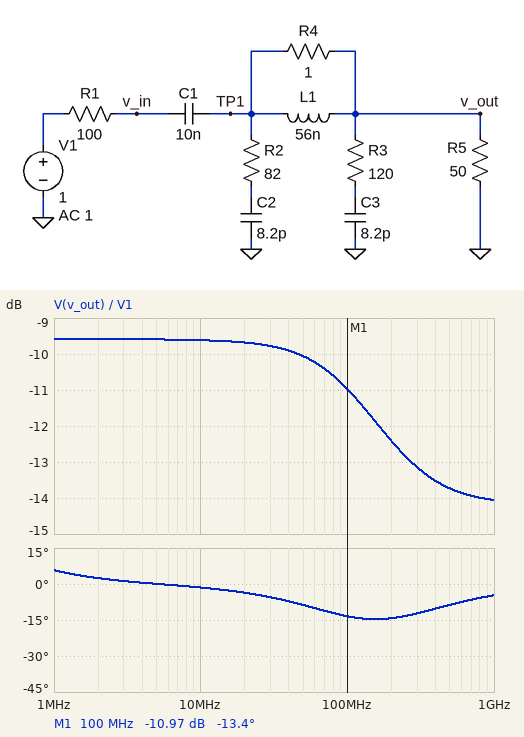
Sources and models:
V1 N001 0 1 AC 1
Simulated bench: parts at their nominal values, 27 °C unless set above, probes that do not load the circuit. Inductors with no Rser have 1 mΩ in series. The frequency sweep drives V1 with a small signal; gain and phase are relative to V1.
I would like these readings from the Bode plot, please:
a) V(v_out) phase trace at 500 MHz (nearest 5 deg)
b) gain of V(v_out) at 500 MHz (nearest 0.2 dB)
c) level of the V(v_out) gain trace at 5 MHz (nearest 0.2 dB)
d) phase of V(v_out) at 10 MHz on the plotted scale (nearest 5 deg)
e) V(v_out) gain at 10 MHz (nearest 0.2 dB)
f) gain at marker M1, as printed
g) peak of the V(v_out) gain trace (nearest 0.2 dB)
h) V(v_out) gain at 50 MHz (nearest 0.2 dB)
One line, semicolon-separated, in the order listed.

-10 deg; -13.8 dB; -9.6 dB; 0 deg; -9.6 dB; -10.97 dB; -9.6 dB; -10.0 dB
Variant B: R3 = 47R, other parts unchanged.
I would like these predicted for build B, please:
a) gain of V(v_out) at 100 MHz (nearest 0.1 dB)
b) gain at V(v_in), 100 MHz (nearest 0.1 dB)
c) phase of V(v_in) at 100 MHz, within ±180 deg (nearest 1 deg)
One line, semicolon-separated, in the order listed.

-10.8 dB; -10.6 dB; -16 deg
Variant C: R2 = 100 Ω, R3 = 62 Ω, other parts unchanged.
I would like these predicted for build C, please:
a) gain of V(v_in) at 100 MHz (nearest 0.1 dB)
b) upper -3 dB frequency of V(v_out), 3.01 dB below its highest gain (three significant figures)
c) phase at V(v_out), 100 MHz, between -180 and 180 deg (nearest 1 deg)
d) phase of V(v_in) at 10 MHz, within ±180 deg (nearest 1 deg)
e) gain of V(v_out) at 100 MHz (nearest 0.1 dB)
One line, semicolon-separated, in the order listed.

-10.7 dB; 208 MHz; -15 deg; -3 deg; -10.9 dB
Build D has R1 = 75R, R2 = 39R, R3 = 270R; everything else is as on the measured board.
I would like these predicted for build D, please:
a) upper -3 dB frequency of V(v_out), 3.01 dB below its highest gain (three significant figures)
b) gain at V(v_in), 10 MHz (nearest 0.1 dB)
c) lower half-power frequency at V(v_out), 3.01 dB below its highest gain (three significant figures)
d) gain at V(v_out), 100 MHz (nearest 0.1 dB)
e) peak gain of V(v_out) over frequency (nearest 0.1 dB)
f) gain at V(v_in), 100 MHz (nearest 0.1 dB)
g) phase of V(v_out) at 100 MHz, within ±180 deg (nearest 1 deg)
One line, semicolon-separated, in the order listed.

340 MHz; -7.9 dB; 126 kHz; -9.0 dB; -8.0 dB; -8.8 dB; -10 deg
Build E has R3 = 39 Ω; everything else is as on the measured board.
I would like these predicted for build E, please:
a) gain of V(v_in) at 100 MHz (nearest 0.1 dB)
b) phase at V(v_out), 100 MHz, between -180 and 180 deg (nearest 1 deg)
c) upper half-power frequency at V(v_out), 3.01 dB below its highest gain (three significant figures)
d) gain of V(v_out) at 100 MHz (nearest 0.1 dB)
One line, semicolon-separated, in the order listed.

-10.5 dB; -16 deg; 211 MHz; -10.7 dB
